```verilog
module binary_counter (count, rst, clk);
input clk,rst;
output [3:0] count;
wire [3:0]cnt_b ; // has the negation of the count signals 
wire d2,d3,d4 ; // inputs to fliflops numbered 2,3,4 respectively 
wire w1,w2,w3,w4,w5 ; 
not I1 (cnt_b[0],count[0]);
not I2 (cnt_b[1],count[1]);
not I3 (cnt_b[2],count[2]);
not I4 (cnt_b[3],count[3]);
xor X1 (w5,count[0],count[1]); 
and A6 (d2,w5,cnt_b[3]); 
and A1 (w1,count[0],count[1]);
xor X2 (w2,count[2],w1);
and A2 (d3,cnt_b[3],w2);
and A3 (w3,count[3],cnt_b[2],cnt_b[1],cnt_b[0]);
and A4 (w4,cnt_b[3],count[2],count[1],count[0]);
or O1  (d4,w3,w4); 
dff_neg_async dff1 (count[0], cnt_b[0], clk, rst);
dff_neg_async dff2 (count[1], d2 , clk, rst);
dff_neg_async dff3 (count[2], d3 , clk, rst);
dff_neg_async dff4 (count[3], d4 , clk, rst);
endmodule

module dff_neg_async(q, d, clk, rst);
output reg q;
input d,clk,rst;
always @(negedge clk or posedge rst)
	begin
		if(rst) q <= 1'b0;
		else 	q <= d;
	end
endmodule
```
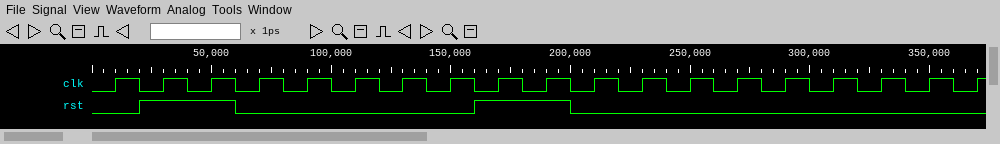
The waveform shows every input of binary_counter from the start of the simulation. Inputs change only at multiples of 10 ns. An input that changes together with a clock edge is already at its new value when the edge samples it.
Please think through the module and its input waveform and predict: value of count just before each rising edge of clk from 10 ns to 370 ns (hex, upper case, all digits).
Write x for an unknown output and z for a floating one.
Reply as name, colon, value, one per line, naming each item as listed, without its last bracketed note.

value of count just before each rising edge of clk from 10 ns to 370 ns: x, 0, 0, 1, 2, 3, 4, 5, 0, 0, 1, 2, 3, 4, 5, 6, 7, 8, 9
